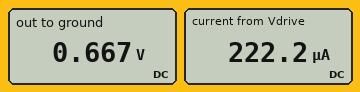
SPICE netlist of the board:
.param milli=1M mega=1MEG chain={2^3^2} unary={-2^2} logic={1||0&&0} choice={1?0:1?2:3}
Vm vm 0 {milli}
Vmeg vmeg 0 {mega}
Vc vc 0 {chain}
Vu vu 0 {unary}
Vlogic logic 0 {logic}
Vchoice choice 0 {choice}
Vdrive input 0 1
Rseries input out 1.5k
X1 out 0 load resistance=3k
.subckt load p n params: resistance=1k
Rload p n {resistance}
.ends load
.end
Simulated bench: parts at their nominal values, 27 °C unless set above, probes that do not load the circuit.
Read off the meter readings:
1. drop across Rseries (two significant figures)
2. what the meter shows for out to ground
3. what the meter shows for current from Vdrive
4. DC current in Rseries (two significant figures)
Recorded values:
330 mV
0.667 V
222.2 µA
220 µA
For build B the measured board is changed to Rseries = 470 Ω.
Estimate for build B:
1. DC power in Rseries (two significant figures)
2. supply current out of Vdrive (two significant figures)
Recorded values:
39 µW
290 µA
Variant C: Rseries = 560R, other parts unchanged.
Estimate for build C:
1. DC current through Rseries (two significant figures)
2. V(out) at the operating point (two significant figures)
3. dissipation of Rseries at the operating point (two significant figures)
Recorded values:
280 µA
840 mV
44 µW
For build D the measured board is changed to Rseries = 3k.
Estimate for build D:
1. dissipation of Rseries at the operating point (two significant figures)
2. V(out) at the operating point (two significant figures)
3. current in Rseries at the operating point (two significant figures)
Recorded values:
83 µW
500 mV
170 µA
